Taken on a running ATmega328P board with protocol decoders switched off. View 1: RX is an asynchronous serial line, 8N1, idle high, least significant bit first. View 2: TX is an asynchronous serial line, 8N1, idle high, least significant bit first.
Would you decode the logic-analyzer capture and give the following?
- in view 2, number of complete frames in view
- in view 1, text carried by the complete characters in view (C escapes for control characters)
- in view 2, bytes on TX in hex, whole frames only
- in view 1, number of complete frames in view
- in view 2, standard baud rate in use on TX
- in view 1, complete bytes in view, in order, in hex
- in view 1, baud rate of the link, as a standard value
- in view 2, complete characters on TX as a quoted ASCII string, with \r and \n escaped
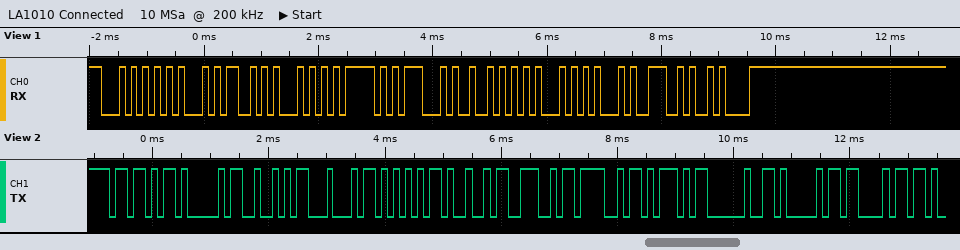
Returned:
12
"TEST_GREEN\n"
0x5B 0x41 0x52 0x44 0x55 0x49 0x4E 0x4F 0x5D 0x20 0x41 0x43
11
9600 baud
54 45 53 54 5F 47 52 45 45 4E 0A
9600 baud
"[ARDUINO] AC"
